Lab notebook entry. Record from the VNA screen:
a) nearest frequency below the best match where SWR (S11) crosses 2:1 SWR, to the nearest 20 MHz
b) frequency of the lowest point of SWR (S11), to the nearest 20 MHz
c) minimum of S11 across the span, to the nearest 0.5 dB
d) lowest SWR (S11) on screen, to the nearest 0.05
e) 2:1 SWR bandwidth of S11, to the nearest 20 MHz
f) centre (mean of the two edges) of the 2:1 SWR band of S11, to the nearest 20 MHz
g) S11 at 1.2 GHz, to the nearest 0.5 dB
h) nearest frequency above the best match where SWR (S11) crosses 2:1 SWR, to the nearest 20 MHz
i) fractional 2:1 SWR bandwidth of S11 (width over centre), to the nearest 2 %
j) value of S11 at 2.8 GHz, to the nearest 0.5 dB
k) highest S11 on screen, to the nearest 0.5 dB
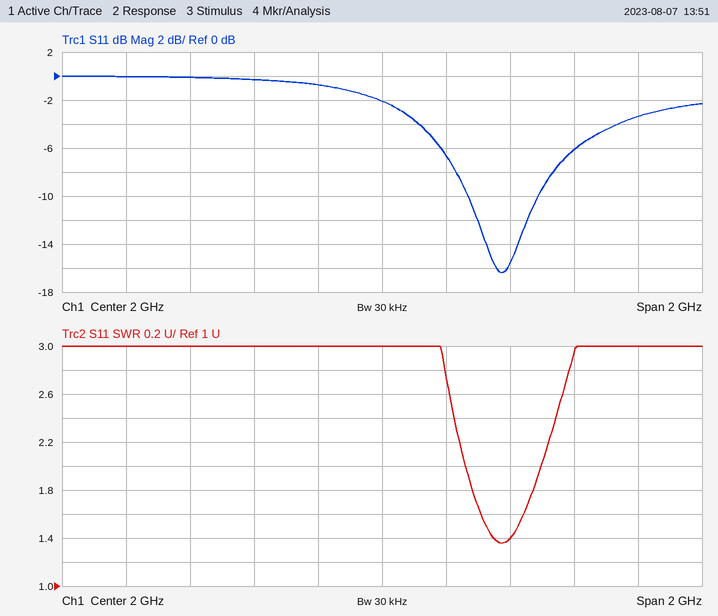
2.26 GHz
2.38 GHz
-16.5 dB
1.35
240 MHz
2.38 GHz
0.0 dB
2.50 GHz
10 %
-3.5 dB
0.0 dB
